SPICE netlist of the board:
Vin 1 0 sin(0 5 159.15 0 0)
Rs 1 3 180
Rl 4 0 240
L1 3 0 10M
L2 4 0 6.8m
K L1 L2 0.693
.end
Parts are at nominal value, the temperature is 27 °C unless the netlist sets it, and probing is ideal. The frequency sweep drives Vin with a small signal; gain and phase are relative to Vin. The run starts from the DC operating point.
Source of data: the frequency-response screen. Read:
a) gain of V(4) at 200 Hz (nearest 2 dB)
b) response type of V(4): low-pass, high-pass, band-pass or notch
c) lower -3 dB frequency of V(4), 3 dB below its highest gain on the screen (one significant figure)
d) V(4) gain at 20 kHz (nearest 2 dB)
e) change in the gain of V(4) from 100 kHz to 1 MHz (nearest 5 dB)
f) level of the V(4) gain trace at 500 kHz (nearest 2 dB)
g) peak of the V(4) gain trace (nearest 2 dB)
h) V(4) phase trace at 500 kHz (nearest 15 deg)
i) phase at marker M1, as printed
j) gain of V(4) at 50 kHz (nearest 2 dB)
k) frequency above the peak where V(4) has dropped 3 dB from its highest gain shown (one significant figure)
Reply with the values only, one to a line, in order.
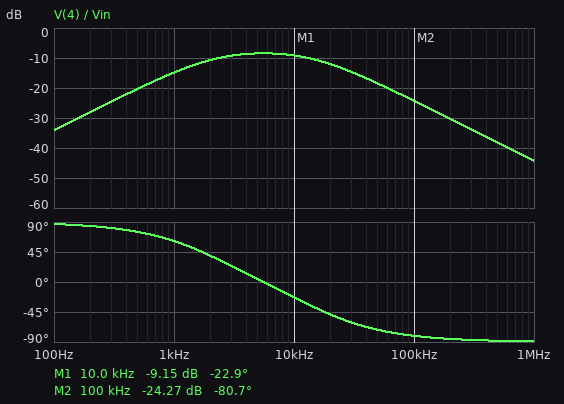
-28 dB
band-pass
2 kHz
-12 dB
-20 dB
-38 dB
-8 dB
-90 deg
-22.9 deg
-18 dB
20 kHz
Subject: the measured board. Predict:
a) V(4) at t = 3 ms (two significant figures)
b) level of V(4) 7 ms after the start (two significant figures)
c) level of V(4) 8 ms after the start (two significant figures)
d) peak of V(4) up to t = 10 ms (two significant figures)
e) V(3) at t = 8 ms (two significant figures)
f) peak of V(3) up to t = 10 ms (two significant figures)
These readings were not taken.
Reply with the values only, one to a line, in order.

-150 mV
130 mV
-9.8 mV
160 mV
-21 mV
280 mV
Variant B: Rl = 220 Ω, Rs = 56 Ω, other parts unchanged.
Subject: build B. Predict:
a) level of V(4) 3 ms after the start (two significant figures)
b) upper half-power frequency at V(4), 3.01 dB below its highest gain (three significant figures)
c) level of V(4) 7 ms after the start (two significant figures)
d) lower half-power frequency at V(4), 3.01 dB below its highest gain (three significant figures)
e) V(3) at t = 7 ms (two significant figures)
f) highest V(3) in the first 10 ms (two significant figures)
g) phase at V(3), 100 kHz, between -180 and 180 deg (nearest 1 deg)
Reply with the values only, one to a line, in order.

-470 mV
12.3 kHz
440 mV
716 Hz
760 mV
880 mV
1 deg
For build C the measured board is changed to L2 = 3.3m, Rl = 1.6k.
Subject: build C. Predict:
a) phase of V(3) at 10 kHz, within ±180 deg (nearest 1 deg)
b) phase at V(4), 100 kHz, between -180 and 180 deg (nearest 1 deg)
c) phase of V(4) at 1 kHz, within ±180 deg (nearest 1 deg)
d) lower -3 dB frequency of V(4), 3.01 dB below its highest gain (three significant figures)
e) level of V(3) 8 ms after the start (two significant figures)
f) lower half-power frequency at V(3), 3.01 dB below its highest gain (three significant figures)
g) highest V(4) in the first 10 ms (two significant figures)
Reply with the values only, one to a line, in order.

16 deg
-32 deg
70 deg
2.71 kHz
-25 mV
2.92 kHz
110 mV
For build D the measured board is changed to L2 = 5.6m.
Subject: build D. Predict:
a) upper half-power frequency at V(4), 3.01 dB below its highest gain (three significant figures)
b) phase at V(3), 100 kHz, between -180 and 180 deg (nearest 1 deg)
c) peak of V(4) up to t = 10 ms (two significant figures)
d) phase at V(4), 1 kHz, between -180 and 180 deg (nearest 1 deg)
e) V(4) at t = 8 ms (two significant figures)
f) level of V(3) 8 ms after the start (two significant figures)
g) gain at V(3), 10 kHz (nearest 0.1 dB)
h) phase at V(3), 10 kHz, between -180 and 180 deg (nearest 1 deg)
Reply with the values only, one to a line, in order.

20.5 kHz
3 deg
140 mV
63 deg
-9.6 mV
-22 mV
-1.5 dB
19 deg
